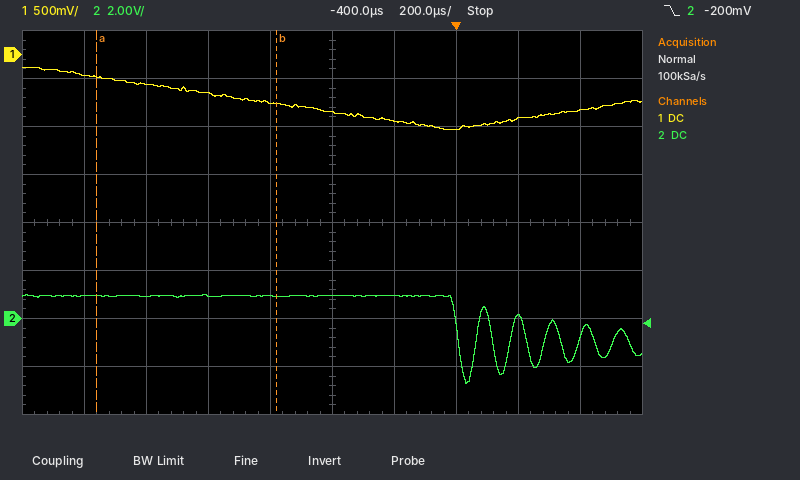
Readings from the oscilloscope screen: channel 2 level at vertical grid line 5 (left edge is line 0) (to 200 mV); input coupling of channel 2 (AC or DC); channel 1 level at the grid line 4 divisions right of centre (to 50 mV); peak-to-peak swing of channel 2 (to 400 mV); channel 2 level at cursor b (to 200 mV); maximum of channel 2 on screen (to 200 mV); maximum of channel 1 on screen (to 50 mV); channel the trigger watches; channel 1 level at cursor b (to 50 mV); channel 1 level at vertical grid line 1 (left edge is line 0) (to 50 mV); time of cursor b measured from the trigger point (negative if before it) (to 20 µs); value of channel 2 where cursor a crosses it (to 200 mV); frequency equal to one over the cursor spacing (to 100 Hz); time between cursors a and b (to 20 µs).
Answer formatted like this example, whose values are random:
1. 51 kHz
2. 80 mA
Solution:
1. 1.0 V
2. DC
3. -600 mV
4. 3.6 V
5. 1.0 V
6. 1.0 V
7. -150 mV
8. channel 2
9. -500 mV
10. -200 mV
11. -580 µs
12. 1.0 V
13. 1.7 kHz
14. 580 µs
